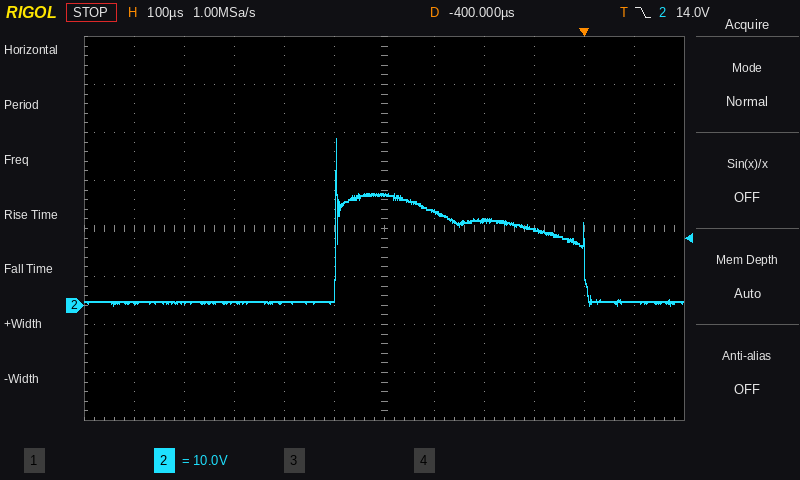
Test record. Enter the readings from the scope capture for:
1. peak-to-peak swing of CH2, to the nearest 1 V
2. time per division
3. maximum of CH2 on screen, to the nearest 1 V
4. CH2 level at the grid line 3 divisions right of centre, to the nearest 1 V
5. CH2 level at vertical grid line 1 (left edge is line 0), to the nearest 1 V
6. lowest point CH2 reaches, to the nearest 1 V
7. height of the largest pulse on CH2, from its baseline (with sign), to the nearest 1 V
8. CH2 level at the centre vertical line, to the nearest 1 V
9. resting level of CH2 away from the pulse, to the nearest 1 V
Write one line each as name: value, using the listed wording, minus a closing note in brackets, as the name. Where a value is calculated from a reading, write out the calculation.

peak-to-peak swing of CH2, to the nearest 1 V: 35 V − (0 V) = 35 V
time per division: 100 µs
maximum of CH2 on screen, to the nearest 1 V: 35 V
CH2 level at the grid line 3 divisions right of centre, to the nearest 1 V: 16 V
CH2 level at vertical grid line 1 (left edge is line 0), to the nearest 1 V: 1 V
lowest point CH2 reaches, to the nearest 1 V: 0 V
height of the largest pulse on CH2, from its baseline (with sign), to the nearest 1 V: 35 V − (1 V) = +34 V
CH2 level at the centre vertical line, to the nearest 1 V: 23 V
resting level of CH2 away from the pulse, to the nearest 1 V: 1 V
